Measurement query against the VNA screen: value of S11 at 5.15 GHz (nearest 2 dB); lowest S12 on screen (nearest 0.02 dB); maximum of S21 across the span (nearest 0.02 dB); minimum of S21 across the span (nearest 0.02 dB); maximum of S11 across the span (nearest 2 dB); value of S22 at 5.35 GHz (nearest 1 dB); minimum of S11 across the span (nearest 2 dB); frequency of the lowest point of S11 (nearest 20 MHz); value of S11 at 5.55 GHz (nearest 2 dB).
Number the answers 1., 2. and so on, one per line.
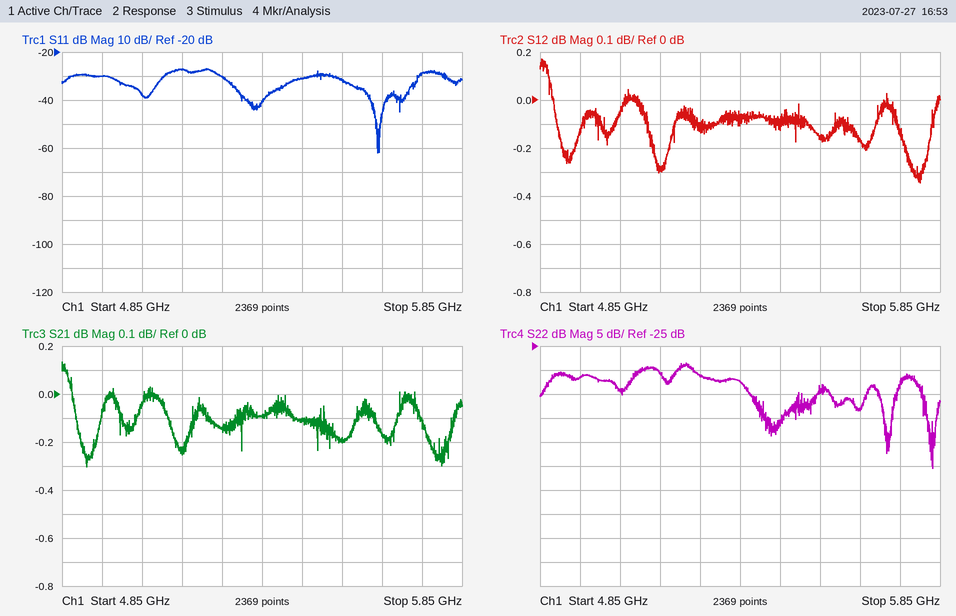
1. -28 dB
2. -0.34 dB
3. 0.14 dB
4. -0.30 dB
5. -26 dB
6. -32 dB
7. -62 dB
8. 5.64 GHz
9. -32 dB
